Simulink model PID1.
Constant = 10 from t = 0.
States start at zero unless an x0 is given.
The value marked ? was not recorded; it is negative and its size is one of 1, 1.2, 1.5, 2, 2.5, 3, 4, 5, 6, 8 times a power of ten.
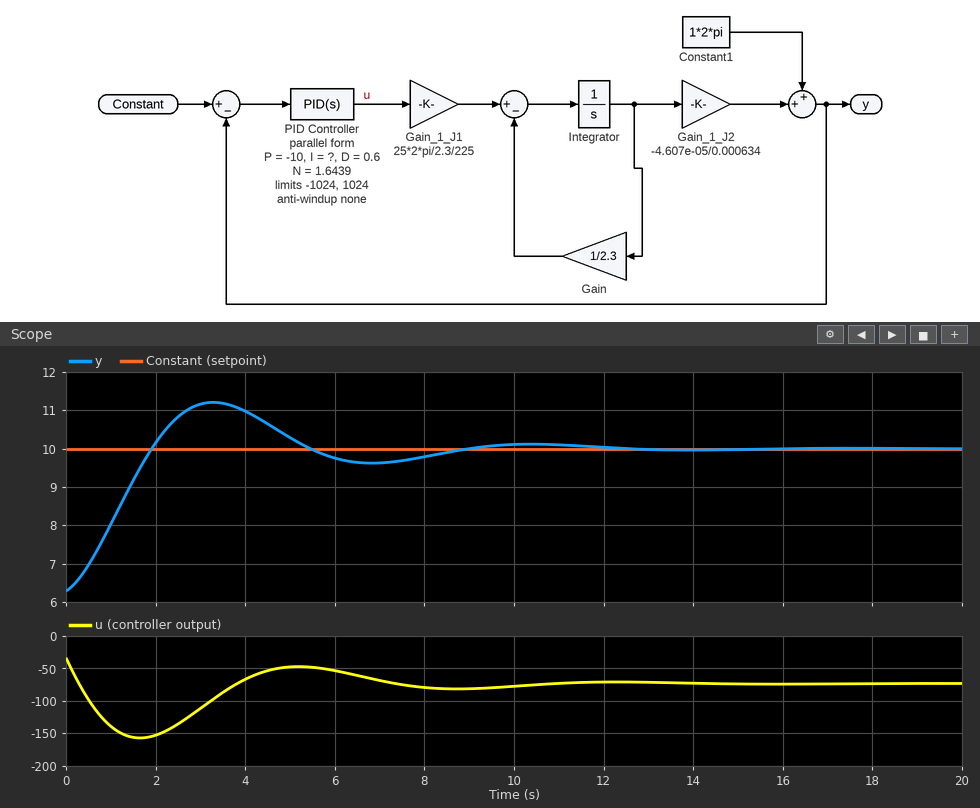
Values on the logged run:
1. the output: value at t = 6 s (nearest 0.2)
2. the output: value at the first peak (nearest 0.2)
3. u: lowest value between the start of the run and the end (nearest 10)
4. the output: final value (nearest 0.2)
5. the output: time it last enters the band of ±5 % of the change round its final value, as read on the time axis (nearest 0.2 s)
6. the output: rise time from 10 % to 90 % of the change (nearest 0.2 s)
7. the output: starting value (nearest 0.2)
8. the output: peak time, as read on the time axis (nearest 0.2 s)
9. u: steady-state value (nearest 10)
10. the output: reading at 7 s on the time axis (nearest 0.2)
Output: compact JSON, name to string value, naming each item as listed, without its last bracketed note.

{"the output: value at t = 6 s": "9.8", "the output: value at the first peak": "11.2", "u: lowest value between the start of the run and the end": "-160", "the output: final value": "10.0", "the output: time it last enters the band of ±5 % of the change round its final value, as read on the time axis": "8.2 s", "the output: rise time from 10 % to 90 % of the change": "1.4 s", "the output: starting value": "6.2", "the output: peak time, as read on the time axis": "3.2 s", "u: steady-state value": "-70", "the output: reading at 7 s on the time axis": "9.6"}
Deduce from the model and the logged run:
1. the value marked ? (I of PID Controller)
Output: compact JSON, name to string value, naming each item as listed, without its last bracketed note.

{"the value marked ?": "-40"}
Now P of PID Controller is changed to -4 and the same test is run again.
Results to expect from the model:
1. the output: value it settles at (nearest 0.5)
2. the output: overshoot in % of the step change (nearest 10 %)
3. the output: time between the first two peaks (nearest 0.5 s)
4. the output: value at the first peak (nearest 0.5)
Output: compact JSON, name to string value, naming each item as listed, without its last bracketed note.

{"the output: value it settles at": "10.0", "the output: overshoot in % of the step change": "40 %", "the output: time between the first two peaks": "7.0 s", "the output: value at the first peak": "11.5"}
